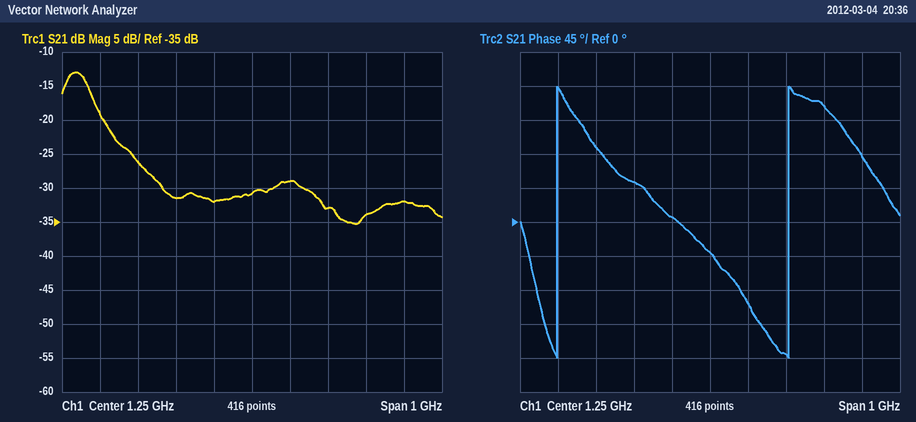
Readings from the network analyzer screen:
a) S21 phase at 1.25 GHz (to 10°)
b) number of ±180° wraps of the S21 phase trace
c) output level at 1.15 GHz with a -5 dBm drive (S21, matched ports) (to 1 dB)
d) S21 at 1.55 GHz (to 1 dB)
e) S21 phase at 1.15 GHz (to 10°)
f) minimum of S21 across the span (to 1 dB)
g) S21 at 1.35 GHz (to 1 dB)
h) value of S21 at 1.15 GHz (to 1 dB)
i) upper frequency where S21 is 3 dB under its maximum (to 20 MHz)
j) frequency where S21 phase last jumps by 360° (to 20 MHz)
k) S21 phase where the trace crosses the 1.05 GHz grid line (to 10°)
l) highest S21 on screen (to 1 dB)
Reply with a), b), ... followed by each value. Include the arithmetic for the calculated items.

a) -40°
b) 2
c) -5 dBm + (-32 dB) = -37 dBm
d) -34 dB
e) 10°
f) -35 dB
g) -29 dB
h) -32 dB
i) 820 MHz
j) 1.46 GHz
k) 50°
l) -13 dB
